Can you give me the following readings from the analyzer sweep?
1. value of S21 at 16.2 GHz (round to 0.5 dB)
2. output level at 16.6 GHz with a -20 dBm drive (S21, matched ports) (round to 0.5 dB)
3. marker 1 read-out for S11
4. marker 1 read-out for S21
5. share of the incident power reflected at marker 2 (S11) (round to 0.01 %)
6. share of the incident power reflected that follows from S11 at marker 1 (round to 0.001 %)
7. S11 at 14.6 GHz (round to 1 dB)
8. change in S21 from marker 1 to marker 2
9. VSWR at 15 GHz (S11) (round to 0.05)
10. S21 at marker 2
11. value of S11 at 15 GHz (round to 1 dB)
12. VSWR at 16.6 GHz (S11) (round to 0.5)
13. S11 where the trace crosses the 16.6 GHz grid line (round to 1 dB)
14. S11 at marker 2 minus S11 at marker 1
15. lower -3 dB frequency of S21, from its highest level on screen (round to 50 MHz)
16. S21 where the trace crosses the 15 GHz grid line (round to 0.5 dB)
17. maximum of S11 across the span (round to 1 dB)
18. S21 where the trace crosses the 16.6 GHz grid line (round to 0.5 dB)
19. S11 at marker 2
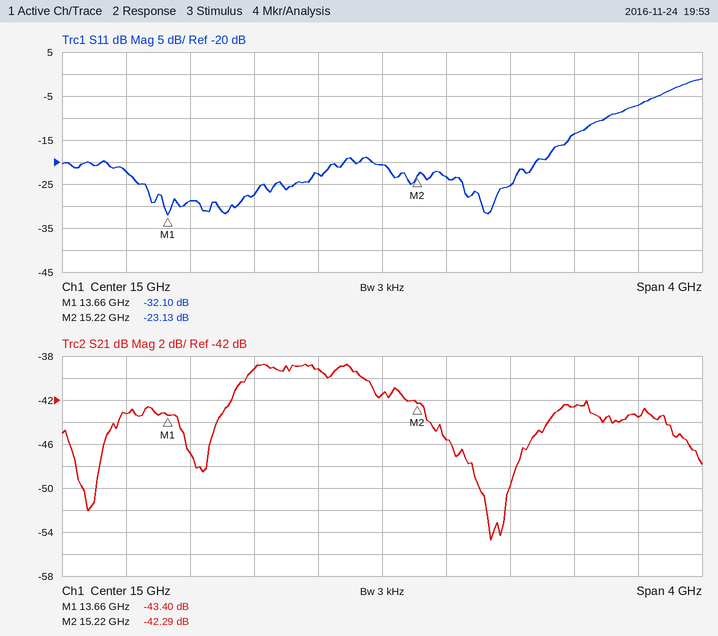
-42.5 dB
-63.5 dBm
-32.10 dB
-43.40 dB
0.49 %
0.062 %
-23 dB
1.11 dB
1.20
-42.29 dB
-21 dB
2.5
-7 dB
8.97 dB
14.05 GHz
-41.5 dB
-1 dB
-43.5 dB
-23.13 dB
